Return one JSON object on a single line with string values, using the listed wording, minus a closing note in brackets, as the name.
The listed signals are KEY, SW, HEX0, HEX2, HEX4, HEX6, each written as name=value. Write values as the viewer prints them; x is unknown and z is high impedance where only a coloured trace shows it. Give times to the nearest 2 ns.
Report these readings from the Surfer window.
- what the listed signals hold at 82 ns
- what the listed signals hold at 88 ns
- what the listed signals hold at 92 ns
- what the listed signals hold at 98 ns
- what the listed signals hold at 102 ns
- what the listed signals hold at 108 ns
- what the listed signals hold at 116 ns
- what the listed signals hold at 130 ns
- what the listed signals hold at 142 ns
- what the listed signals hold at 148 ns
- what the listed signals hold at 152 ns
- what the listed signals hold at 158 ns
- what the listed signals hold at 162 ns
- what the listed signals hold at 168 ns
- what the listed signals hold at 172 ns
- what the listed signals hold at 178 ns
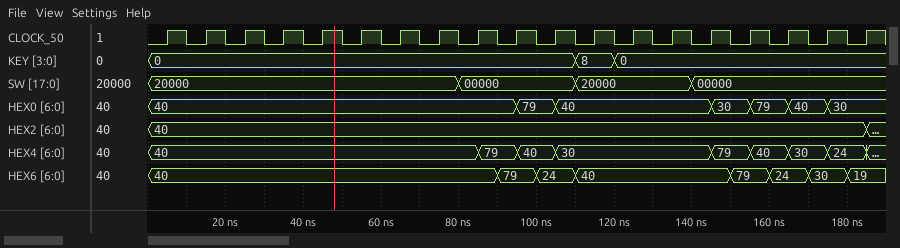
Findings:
{"what the listed signals hold at 82 ns": "KEY=0, SW=00000, HEX0=40, HEX2=40, HEX4=40, HEX6=40", "what the listed signals hold at 88 ns": "KEY=0, SW=00000, HEX0=40, HEX2=40, HEX4=79, HEX6=40", "what the listed signals hold at 92 ns": "KEY=0, SW=00000, HEX0=40, HEX2=40, HEX4=79, HEX6=79", "what the listed signals hold at 98 ns": "KEY=0, SW=00000, HEX0=79, HEX2=40, HEX4=40, HEX6=79", "what the listed signals hold at 102 ns": "KEY=0, SW=00000, HEX0=79, HEX2=40, HEX4=40, HEX6=24", "what the listed signals hold at 108 ns": "KEY=0, SW=00000, HEX0=40, HEX2=40, HEX4=30, HEX6=24", "what the listed signals hold at 116 ns": "KEY=8, SW=20000, HEX0=40, HEX2=40, HEX4=30, HEX6=40", "what the listed signals hold at 130 ns": "KEY=0, SW=20000, HEX0=40, HEX2=40, HEX4=30, HEX6=40", "what the listed signals hold at 142 ns": "KEY=0, SW=00000, HEX0=40, HEX2=40, HEX4=30, HEX6=40", "what the listed signals hold at 148 ns": "KEY=0, SW=00000, HEX0=30, HEX2=40, HEX4=79, HEX6=40", "what the listed signals hold at 152 ns": "KEY=0, SW=00000, HEX0=30, HEX2=40, HEX4=79, HEX6=79", "what the listed signals hold at 158 ns": "KEY=0, SW=00000, HEX0=79, HEX2=40, HEX4=40, HEX6=79", "what the listed signals hold at 162 ns": "KEY=0, SW=00000, HEX0=79, HEX2=40, HEX4=40, HEX6=24", "what the listed signals hold at 168 ns": "KEY=0, SW=00000, HEX0=40, HEX2=40, HEX4=30, HEX6=24", "what the listed signals hold at 172 ns": "KEY=0, SW=00000, HEX0=40, HEX2=40, HEX4=30, HEX6=30", "what the listed signals hold at 178 ns": "KEY=0, SW=00000, HEX0=30, HEX2=40, HEX4=24, HEX6=30"}
